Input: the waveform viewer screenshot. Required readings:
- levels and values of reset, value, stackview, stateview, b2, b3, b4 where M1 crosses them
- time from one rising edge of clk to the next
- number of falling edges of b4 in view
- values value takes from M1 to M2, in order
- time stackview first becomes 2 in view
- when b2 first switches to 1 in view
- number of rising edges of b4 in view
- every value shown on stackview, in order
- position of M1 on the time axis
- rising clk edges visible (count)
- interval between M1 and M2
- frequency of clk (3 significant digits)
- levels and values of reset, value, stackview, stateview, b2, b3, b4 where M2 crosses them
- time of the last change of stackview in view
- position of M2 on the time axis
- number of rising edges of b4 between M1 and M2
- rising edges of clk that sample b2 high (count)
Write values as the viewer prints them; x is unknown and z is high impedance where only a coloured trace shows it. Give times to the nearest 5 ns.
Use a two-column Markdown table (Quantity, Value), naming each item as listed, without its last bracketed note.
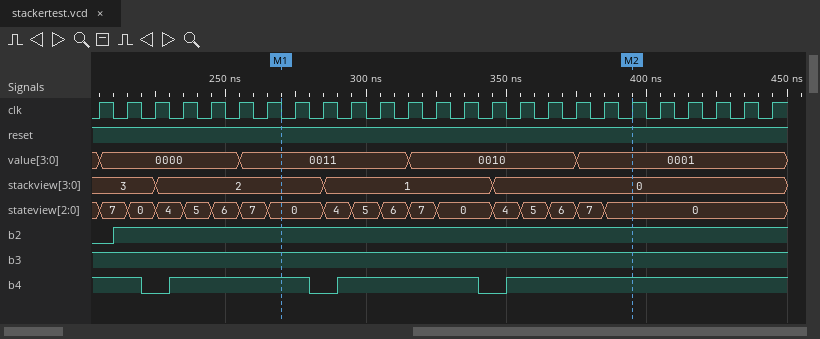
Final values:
| Quantity | Value |
|---|---|
| levels and values of reset, value, stackview, stateview, b2, b3, b4 where M1 crosses them | reset=1, value=0011, stackview=2, stateview=0, b2=1, b3=1, b4=1 |
| time from one rising edge of clk to the next | 10 ns |
| number of falling edges of b4 in view | 3 |
| values value takes from M1 to M2, in order | 0011, 0010, 0001 |
| time stackview first becomes 2 in view | 225 ns |
| when b2 first switches to 1 in view | 210 ns |
| number of rising edges of b4 in view | 3 |
| every value shown on stackview, in order | 3, 2, 1, 0 |
| position of M1 on the time axis | 270 ns |
| rising clk edges visible | 25 |
| interval between M1 and M2 | 125 ns |
| frequency of clk | 100 MHz |
| levels and values of reset, value, stackview, stateview, b2, b3, b4 where M2 crosses them | reset=1, value=0001, stackview=0, stateview=0, b2=1, b3=1, b4=1 |
| time of the last change of stackview in view | 345 ns |
| position of M2 on the time axis | 395 ns |
| number of rising edges of b4 between M1 and M2 | 2 |
| rising edges of clk that sample b2 high | 24 |
